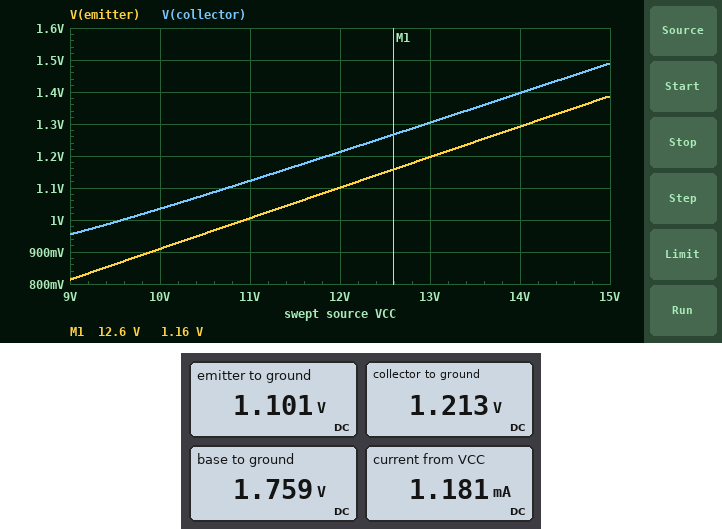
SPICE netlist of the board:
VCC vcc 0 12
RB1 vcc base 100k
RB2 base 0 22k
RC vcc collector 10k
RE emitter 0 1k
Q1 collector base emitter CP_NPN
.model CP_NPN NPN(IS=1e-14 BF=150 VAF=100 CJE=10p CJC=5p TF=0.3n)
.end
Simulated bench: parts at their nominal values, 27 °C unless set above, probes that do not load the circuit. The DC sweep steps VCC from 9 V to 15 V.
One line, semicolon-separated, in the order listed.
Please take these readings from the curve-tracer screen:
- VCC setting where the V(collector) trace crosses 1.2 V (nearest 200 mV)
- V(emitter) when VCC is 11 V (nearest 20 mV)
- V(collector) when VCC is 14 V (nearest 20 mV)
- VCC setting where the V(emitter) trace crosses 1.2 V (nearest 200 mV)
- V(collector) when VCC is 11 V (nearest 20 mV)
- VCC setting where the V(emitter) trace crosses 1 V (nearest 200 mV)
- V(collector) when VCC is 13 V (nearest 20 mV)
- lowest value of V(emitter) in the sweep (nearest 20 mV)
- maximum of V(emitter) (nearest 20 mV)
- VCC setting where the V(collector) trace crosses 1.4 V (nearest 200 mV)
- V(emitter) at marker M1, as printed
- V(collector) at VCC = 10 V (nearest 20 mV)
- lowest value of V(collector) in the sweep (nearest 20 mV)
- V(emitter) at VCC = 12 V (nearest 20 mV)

11.8 V; 1.00 V; 1.40 V; 13.0 V; 1.12 V; 11.0 V; 1.30 V; 820 mV; 1.38 V; 14.0 V; 1.16 V; 1.04 V; 960 mV; 1.10 V
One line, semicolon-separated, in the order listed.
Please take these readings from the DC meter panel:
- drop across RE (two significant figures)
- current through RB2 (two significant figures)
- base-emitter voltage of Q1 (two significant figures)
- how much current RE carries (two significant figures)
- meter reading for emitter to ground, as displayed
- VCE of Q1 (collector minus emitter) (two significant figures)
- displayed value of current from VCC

1.1 V; 80 µA; 660 mV; 1.1 mA; 1.101 V; 110 mV; 1.181 mA
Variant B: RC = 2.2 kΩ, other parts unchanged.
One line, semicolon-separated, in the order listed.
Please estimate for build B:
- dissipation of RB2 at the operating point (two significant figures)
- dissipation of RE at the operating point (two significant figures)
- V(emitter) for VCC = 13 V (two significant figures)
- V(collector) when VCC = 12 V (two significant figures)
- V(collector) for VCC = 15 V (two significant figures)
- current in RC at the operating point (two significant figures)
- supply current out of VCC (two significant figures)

180 µW; 1.8 mW; 1.5 V; 9.0 V; 11 V; 1.3 mA; 1.4 mA
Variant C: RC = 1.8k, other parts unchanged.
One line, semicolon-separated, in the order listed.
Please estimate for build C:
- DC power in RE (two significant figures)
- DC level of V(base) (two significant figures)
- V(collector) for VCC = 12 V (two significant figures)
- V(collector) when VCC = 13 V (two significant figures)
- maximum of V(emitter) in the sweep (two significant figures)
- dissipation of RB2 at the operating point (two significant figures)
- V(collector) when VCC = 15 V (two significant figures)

1.8 mW; 2.0 V; 9.6 V; 10 V; 1.8 V; 180 µW; 12 V
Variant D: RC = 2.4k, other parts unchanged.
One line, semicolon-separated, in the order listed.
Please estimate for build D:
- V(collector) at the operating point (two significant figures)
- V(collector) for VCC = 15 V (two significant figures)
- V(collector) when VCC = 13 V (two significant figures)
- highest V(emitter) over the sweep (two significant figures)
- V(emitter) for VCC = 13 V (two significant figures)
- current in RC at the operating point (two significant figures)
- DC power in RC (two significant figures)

8.8 V; 11 V; 9.4 V; 1.8 V; 1.5 V; 1.3 mA; 4.3 mW
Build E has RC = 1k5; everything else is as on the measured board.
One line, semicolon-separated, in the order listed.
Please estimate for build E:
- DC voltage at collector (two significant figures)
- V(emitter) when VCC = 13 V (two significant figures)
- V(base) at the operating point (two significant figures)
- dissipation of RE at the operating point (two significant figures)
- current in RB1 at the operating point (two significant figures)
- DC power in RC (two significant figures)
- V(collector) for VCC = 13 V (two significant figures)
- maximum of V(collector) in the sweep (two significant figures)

10 V; 1.5 V; 2.0 V; 1.8 mW; 100 µA; 2.7 mW; 11 V; 12 V
